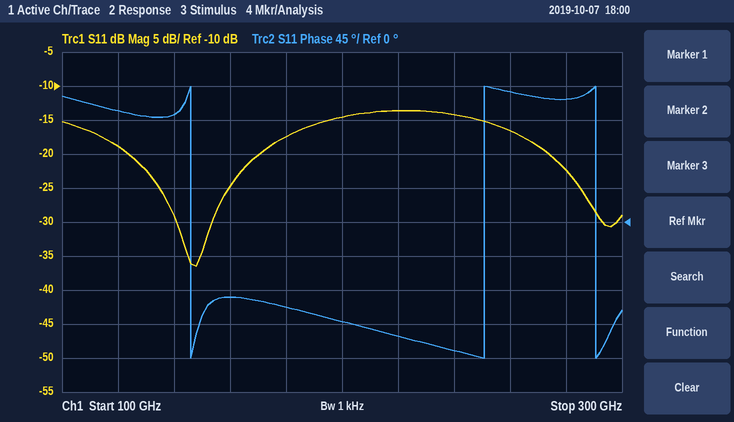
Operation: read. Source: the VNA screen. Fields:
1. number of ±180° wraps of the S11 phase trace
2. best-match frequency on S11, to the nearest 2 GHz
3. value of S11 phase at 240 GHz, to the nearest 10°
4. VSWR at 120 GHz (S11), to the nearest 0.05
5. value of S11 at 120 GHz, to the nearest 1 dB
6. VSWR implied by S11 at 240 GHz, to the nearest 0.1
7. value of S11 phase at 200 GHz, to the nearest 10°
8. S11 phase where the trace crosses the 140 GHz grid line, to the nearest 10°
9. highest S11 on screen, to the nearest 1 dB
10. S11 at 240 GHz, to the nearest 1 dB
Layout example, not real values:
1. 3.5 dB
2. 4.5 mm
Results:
1. 3
2. 148 GHz
3. -170°
4. 1.25
5. -19 dB
6. 1.5
7. -130°
8. 140°
9. -14 dB
10. -14 dB
